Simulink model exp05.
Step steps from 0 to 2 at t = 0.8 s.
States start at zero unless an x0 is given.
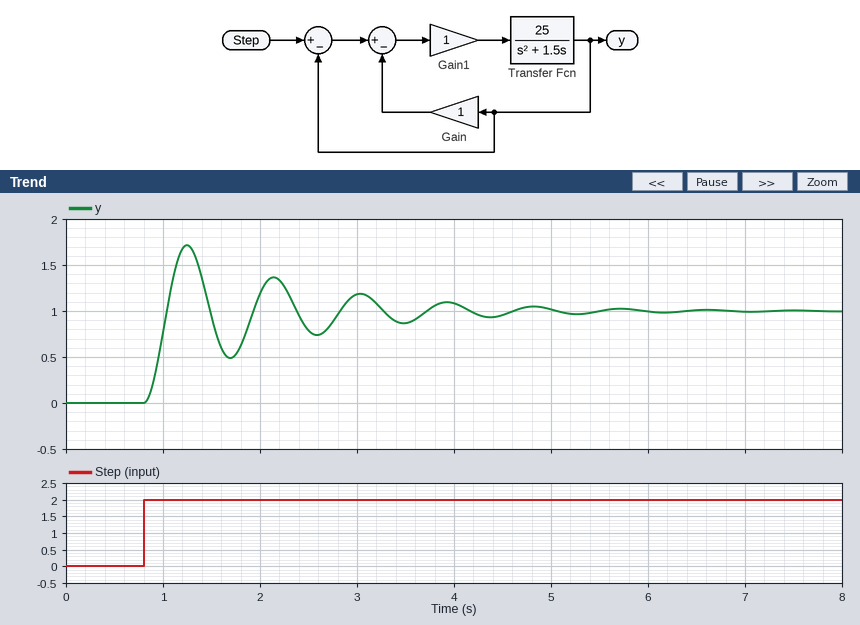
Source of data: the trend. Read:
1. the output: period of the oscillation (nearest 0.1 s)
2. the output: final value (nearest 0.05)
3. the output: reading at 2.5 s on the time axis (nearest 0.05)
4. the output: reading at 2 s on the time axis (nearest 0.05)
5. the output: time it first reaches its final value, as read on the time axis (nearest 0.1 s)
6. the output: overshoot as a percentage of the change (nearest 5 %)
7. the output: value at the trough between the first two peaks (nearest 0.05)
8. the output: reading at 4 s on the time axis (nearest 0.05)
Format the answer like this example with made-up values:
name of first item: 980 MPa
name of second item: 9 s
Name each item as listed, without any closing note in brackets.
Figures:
the output: period of the oscillation: 0.9 s
the output: final value: 1.00
the output: reading at 2.5 s on the time axis: 0.80
the output: reading at 2 s on the time axis: 1.20
the output: time it first reaches its final value, as read on the time axis: 1.0 s
the output: overshoot as a percentage of the change: 70 %
the output: value at the trough between the first two peaks: 0.50
the output: reading at 4 s on the time axis: 1.10
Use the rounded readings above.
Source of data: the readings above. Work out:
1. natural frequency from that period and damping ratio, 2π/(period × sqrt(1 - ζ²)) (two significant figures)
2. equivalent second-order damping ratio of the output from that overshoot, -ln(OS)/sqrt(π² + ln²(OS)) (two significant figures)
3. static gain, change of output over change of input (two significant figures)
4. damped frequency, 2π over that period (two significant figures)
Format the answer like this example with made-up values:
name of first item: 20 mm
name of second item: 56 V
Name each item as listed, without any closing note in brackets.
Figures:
natural frequency from that period and damping ratio, 2π/(period × sqrt(1 - ζ²)): 7.0 rad/s
equivalent second-order damping ratio of the output from that overshoot, -ln(OS)/sqrt(π² + ln²(OS)): 0.11
static gain, change of output over change of input: 0.50
damped frequency, 2π over that period: 7.0 rad/s
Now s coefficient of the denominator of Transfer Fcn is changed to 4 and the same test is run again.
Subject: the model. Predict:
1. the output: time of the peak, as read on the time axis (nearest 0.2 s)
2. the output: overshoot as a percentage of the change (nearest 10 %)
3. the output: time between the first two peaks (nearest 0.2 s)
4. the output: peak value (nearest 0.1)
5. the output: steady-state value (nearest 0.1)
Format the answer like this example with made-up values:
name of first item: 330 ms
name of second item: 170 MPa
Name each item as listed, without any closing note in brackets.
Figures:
the output: time of the peak, as read on the time axis: 1.2 s
the output: overshoot as a percentage of the change: 40 %
the output: time between the first two peaks: 1.0 s
the output: peak value: 1.4
the output: steady-state value: 1.0
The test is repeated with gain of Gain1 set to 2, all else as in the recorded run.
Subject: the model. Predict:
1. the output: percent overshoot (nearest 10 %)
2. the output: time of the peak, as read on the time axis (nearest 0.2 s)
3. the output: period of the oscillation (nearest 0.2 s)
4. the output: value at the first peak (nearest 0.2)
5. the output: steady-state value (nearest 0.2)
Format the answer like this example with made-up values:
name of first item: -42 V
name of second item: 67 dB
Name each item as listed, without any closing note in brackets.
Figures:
the output: percent overshoot: 80 %
the output: time of the peak, as read on the time axis: 1.2 s
the output: period of the oscillation: 0.6 s
the output: value at the first peak: 1.8
the output: steady-state value: 1.0
